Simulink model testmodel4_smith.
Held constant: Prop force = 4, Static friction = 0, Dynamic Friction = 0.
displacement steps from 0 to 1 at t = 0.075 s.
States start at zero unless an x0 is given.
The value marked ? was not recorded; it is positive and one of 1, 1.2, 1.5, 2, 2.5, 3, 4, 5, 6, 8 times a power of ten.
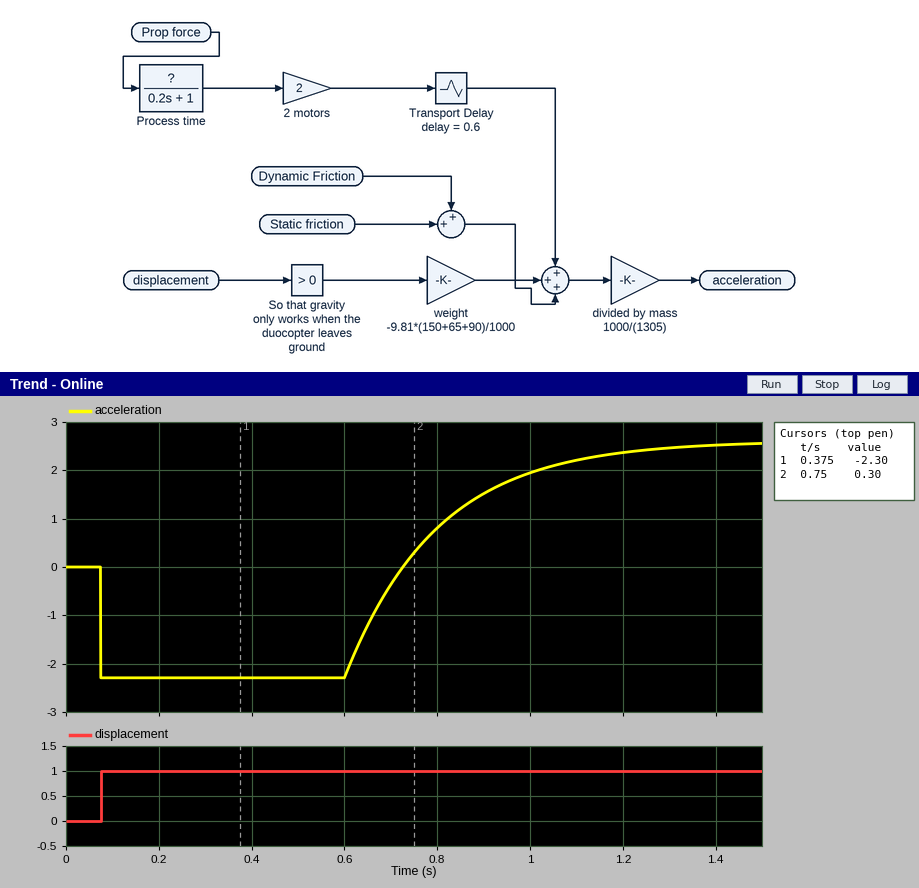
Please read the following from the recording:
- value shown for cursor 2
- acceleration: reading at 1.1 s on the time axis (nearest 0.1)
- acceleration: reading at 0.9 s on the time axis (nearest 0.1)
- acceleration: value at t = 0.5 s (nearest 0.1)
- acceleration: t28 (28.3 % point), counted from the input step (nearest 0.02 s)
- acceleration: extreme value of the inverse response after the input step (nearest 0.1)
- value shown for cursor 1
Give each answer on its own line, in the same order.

0.30
2.2
1.5
-2.3
0.72 s
-2.3
-2.30
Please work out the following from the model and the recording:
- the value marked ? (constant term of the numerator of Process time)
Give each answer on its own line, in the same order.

0.8
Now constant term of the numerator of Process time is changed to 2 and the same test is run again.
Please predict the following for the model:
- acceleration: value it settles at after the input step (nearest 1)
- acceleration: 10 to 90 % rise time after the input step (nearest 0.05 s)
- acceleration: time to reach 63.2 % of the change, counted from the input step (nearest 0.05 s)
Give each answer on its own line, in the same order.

10
0.45 s
0.75 s
